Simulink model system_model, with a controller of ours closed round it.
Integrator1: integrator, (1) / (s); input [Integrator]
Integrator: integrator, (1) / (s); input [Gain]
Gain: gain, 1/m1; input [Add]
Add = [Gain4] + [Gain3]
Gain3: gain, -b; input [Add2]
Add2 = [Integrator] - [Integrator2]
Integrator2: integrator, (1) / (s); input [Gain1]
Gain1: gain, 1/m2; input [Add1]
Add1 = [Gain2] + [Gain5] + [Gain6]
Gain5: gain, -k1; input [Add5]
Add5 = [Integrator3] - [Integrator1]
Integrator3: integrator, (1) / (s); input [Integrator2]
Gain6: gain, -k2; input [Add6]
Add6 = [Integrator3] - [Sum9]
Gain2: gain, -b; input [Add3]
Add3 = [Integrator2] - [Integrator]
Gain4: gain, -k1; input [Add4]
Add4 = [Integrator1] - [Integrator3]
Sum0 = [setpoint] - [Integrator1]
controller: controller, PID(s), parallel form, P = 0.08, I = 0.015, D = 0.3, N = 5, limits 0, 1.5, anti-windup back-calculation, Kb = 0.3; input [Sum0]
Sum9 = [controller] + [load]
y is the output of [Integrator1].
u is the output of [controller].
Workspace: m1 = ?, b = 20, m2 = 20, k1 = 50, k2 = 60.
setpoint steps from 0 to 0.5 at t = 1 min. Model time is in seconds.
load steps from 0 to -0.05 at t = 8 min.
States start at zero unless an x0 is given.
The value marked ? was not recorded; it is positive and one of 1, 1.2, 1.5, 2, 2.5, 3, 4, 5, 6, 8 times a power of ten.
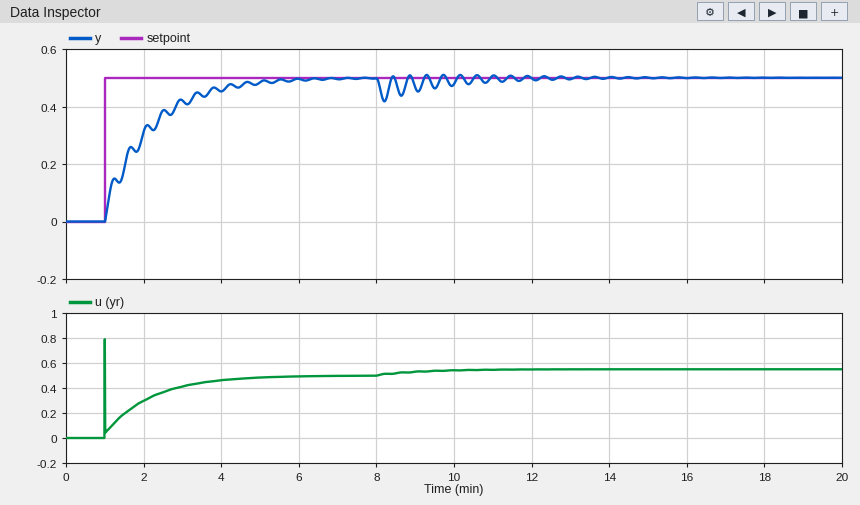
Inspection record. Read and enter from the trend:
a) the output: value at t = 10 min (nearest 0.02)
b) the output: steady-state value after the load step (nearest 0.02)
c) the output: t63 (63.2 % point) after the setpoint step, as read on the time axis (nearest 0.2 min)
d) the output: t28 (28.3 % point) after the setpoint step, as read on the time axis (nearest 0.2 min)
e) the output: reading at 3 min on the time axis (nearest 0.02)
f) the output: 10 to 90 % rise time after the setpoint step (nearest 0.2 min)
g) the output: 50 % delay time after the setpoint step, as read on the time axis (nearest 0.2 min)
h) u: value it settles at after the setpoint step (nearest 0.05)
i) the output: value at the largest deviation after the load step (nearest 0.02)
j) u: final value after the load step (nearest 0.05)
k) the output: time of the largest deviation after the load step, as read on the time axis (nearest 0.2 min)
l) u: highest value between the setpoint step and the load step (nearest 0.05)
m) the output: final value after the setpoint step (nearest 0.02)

0.48
0.50
2.0 min
1.2 min
0.42
2.6 min
1.6 min
0.50
0.42
0.55
8.2 min
0.80
0.50
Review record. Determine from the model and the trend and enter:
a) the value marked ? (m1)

500
